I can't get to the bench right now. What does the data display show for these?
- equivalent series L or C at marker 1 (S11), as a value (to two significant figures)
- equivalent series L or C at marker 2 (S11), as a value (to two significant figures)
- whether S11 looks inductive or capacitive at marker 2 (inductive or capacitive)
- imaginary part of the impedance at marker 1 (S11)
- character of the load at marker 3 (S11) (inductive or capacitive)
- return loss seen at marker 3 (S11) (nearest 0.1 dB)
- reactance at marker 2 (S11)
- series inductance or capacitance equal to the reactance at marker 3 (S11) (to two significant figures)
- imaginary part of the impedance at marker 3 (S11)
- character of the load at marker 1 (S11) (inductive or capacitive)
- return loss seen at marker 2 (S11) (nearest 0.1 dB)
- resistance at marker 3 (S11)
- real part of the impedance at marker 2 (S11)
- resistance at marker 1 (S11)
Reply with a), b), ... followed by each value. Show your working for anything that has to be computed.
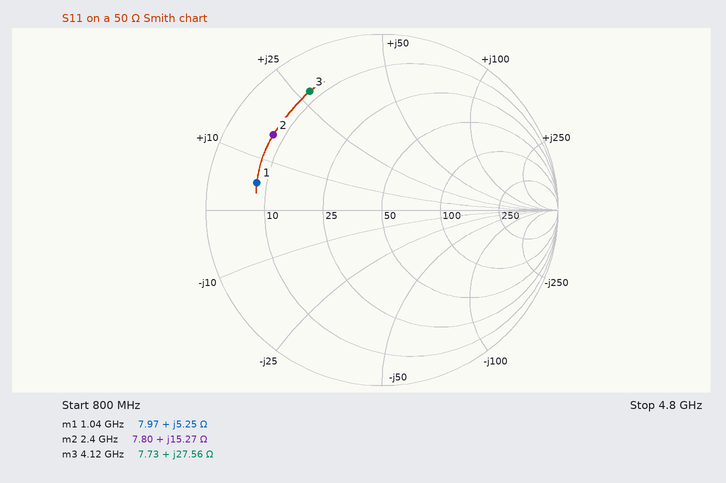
a) L = 5.25 Ω/(2π × 1.04 GHz) ≈ 803 pH, so 800 pH to two significant figures
b) L = 15.27 Ω/(2π × 2.4 GHz) ≈ 1.0 nH
c) inductive
d) +5.25 Ω
e) inductive
f) 2.1 dB
g) +15.27 Ω
h) L = 27.56 Ω/(2π × 4.12 GHz) ≈ 1.1 nH
i) +27.56 Ω
j) inductive
k) 2.5 dB
l) 7.73 Ω
m) 7.80 Ω
n) 7.97 Ω
